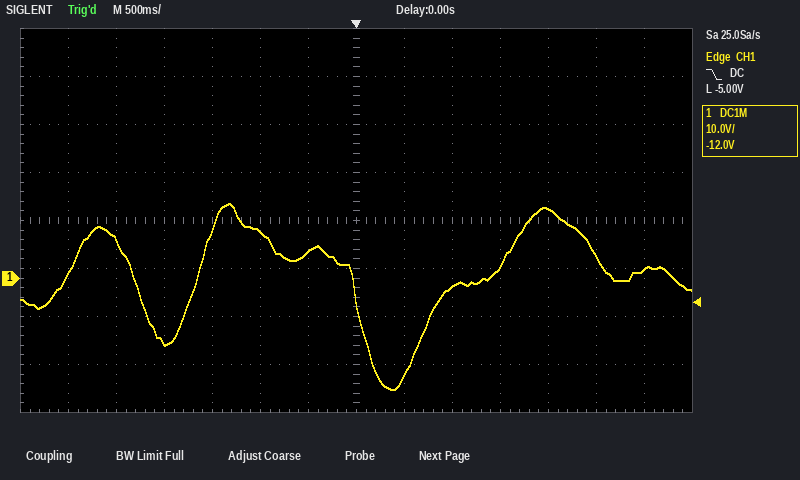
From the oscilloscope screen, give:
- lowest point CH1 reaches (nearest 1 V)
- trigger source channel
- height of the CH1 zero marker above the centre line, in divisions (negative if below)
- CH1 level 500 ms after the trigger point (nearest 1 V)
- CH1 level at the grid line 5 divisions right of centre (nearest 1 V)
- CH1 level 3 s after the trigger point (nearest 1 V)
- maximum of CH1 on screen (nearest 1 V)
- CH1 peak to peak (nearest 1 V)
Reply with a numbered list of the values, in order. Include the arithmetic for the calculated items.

1. -23 V
2. CH1
3. -1.2 div
4. -20 V
5. 5 V
6. 2 V
7. 16 V
8. 16 V − (-23 V) = 39 V
